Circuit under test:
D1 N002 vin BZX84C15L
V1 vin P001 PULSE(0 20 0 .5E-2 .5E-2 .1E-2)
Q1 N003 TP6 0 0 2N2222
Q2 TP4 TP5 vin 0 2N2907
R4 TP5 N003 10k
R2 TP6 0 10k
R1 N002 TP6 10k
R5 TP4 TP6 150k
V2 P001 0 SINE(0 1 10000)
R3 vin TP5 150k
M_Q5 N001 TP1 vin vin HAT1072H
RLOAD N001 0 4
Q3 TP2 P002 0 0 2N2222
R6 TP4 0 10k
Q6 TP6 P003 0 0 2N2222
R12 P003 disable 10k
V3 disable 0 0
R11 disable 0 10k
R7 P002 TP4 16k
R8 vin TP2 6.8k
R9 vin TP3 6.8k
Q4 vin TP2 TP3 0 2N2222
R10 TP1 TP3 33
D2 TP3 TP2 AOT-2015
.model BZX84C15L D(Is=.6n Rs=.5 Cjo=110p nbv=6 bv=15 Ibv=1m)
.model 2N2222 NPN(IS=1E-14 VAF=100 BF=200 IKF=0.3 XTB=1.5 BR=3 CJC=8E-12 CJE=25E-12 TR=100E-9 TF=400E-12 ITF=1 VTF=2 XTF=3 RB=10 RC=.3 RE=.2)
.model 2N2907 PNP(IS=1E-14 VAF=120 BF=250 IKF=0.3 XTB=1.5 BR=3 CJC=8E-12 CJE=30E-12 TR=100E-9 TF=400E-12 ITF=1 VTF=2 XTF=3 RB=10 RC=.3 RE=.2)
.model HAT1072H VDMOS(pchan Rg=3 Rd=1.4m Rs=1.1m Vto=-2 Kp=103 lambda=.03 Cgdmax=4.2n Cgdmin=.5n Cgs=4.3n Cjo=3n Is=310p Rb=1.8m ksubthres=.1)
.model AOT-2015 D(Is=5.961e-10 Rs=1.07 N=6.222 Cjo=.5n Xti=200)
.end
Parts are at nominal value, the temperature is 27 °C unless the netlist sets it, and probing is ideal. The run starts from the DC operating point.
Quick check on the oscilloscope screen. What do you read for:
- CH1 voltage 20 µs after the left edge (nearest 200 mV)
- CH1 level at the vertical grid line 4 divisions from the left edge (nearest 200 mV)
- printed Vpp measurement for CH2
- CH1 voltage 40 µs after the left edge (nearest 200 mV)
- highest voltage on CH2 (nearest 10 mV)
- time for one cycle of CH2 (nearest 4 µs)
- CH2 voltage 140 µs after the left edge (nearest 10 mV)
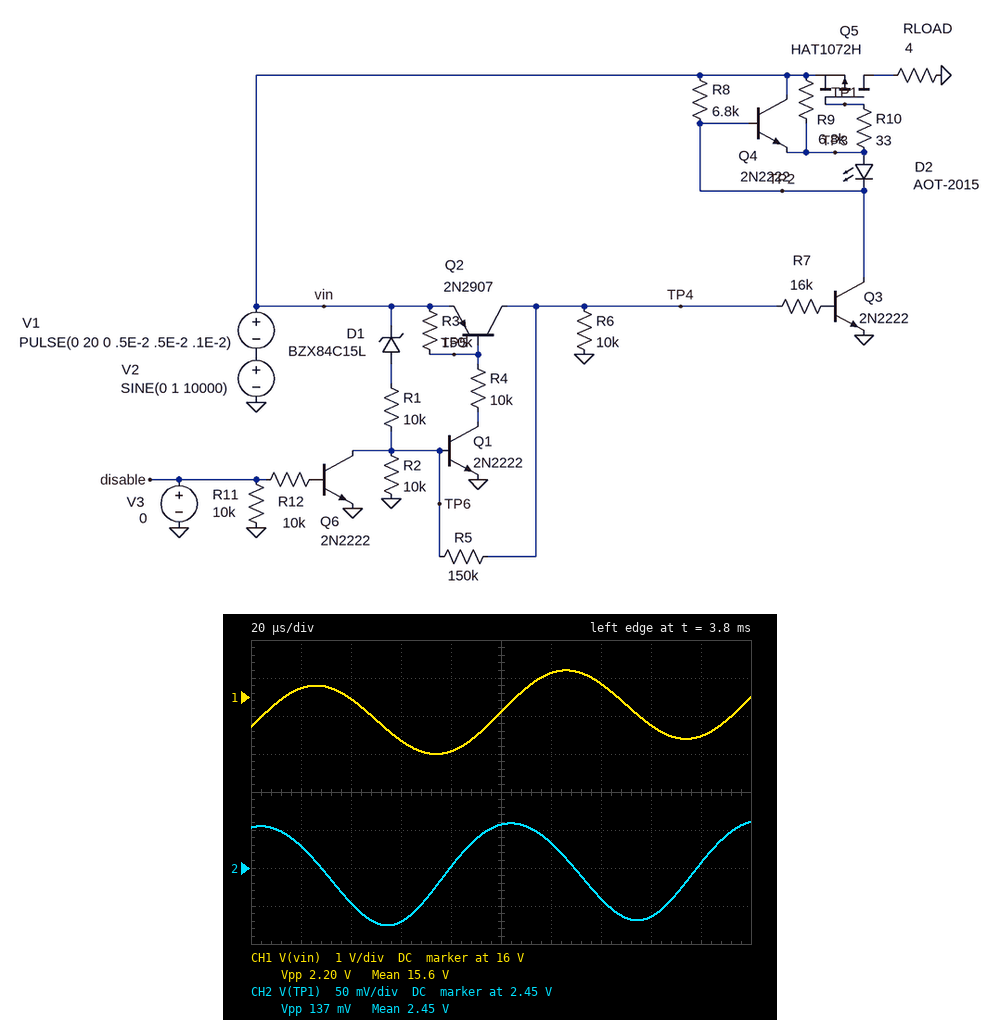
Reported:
16.2 V
14.6 V
137 mV
16.0 V
2.51 V
100 µs
2.41 V
